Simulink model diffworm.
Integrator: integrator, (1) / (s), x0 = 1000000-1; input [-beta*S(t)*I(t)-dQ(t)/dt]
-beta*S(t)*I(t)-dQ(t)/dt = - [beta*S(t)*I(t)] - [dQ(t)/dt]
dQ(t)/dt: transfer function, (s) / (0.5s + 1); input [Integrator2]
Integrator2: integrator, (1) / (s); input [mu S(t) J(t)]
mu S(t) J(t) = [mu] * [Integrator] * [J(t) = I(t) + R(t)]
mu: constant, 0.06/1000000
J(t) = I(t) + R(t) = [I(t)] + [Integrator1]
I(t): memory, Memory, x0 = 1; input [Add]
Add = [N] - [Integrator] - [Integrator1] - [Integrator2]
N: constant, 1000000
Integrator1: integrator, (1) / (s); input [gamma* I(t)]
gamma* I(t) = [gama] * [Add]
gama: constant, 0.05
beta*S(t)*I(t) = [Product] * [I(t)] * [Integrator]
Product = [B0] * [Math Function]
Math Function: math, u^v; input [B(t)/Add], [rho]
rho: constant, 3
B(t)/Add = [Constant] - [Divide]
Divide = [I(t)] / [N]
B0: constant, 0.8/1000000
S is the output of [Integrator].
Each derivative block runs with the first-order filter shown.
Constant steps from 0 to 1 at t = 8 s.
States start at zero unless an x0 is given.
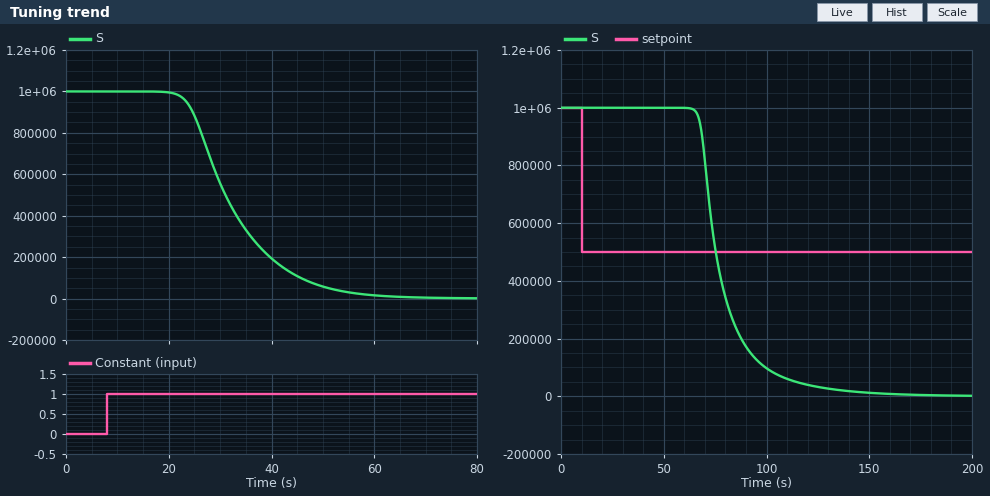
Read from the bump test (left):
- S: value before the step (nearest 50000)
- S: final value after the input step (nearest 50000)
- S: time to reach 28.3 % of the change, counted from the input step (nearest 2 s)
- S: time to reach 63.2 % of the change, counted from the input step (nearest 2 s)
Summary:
1000000
0
20 s
26 s
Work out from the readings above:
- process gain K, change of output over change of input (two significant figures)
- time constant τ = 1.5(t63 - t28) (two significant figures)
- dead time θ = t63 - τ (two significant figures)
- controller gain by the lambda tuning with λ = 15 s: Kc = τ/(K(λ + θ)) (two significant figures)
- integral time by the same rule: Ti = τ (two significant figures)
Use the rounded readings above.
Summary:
-1000000
9.0 s
17 s
-0.00000028
9.0 s
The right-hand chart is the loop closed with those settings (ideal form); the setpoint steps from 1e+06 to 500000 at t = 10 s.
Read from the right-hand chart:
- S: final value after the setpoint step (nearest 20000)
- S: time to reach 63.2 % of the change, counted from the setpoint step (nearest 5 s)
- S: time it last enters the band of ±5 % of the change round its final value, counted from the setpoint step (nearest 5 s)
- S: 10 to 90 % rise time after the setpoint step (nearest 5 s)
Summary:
0
70 s
105 s
30 s
